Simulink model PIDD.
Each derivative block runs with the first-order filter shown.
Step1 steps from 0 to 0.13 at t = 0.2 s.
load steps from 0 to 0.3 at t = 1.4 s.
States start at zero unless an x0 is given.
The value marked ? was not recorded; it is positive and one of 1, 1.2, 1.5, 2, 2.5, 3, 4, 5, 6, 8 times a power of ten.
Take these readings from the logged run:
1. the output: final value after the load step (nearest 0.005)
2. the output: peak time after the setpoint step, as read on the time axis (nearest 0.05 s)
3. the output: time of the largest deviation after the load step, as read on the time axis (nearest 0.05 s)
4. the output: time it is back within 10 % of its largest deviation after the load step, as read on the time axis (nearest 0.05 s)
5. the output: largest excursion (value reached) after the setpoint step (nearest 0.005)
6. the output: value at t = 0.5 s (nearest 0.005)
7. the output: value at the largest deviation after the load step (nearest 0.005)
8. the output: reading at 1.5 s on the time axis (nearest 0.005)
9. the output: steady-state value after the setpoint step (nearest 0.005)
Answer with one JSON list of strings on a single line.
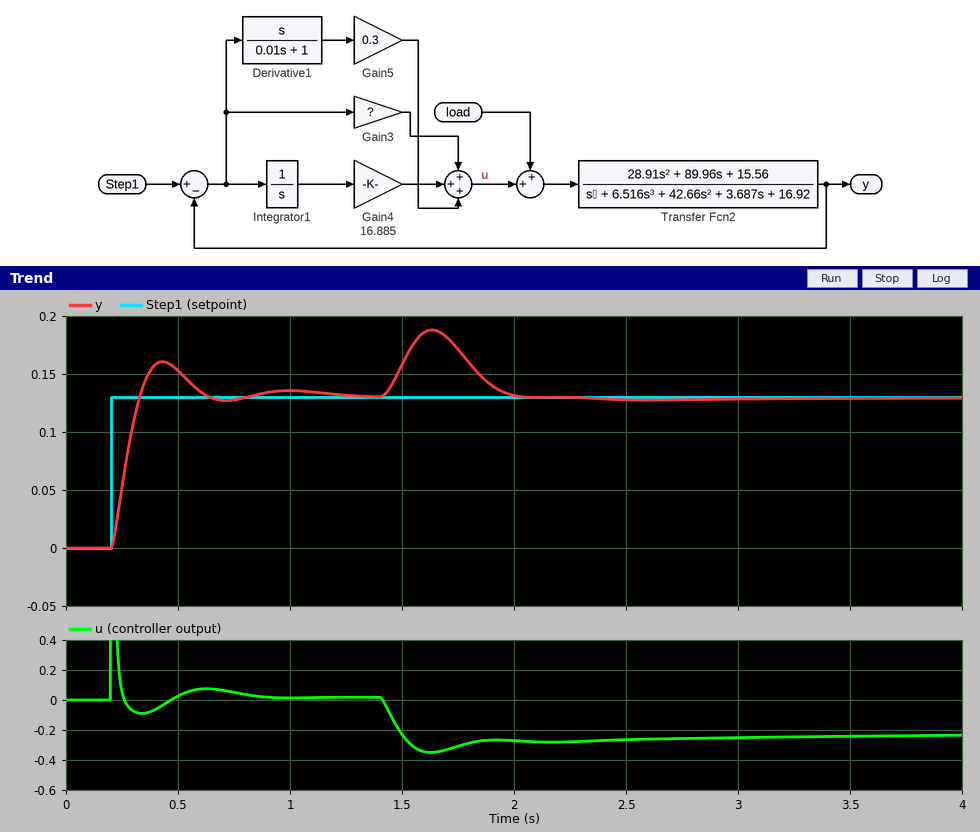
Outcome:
["0.130", "0.45 s", "1.65 s", "1.95 s", "0.160", "0.155", "0.190", "0.160", "0.130"]
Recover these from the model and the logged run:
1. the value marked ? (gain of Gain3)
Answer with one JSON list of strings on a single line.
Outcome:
["4"]
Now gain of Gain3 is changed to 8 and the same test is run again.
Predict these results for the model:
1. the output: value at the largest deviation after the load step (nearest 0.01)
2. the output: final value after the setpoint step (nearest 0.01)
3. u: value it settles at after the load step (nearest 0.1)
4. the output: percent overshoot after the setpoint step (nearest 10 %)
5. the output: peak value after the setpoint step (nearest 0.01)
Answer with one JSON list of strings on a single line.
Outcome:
["0.17", "0.13", "-0.2", "30 %", "0.17"]
